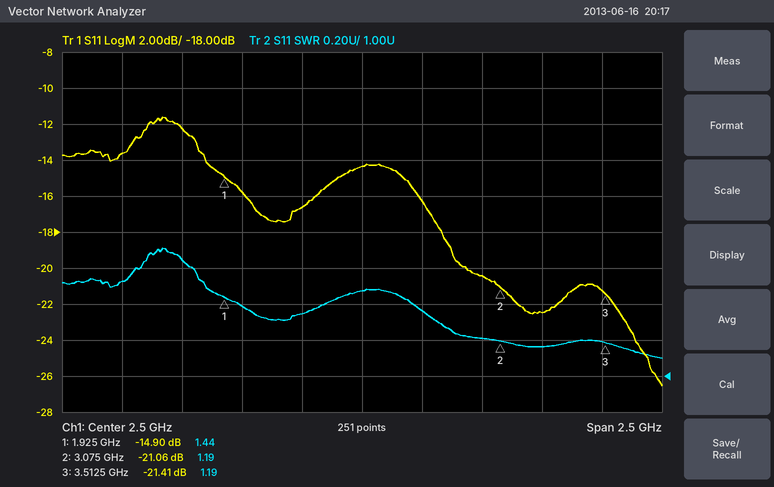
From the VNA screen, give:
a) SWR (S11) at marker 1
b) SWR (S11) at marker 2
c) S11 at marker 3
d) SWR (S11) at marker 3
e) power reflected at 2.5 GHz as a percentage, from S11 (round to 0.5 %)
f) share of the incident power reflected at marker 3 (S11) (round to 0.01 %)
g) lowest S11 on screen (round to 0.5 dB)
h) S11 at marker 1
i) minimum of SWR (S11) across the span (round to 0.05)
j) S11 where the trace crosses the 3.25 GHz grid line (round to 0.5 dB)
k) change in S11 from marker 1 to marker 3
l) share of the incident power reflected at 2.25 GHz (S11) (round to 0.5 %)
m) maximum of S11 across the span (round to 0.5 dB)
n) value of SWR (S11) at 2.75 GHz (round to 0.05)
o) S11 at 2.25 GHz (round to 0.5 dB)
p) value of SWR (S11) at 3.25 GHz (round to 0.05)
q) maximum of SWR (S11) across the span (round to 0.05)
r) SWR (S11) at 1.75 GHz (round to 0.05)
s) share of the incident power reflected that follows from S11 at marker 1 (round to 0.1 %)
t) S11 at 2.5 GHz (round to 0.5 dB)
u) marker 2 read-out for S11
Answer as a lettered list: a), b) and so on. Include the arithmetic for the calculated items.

a) 1.44
b) 1.19
c) -21.41 dB
d) 1.19
e) 10^(-14.5/10) ≈ 3.5 %
f) 10^(-21.41/10) ≈ 0.72 %
g) -26.5 dB
h) -14.90 dB
i) 1.10
j) -22.5 dB
k) -21.41 − (-14.9) = -6.51 dB
l) 10^(-16.5/10) ≈ 2.24 %, so 2.0 % to the nearest 0.5 %
m) -11.5 dB
n) 1.35
o) -16.5 dB
p) 1.15
q) 1.70
r) 1.65
s) 10^(-14.9/10) ≈ 3.2 %
t) -14.5 dB
u) -21.06 dB
